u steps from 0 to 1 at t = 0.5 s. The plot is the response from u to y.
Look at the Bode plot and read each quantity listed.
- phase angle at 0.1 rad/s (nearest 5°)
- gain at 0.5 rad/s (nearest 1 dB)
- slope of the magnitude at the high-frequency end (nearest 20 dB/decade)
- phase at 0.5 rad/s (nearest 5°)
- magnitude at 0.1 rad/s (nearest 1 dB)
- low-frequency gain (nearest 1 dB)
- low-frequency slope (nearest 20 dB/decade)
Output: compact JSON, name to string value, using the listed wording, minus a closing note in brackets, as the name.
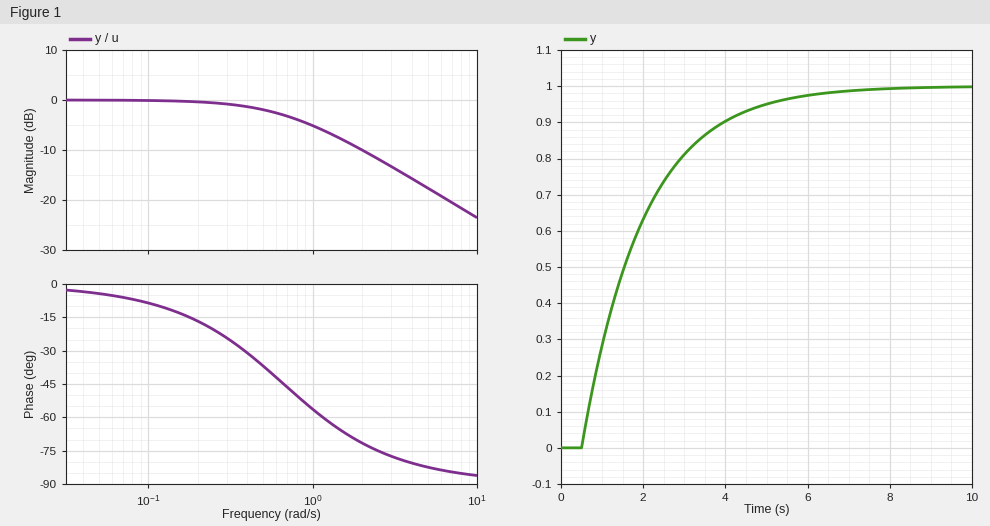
{"phase angle at 0.1 rad/s": "-10°", "gain at 0.5 rad/s": "-2 dB", "slope of the magnitude at the high-frequency end": "-20 dB/decade", "phase at 0.5 rad/s": "-35°", "magnitude at 0.1 rad/s": "0 dB", "low-frequency gain": "0 dB", "low-frequency slope": "0 dB/decade"}
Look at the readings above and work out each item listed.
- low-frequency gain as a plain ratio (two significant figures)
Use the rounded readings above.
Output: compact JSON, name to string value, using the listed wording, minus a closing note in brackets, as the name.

{"low-frequency gain as a plain ratio": "1.0"}
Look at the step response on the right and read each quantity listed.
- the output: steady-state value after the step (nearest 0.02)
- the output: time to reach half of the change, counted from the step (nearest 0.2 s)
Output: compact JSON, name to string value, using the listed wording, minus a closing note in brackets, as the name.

{"the output: steady-state value after the step": "1.00", "the output: time to reach half of the change, counted from the step": "1.0 s"}
